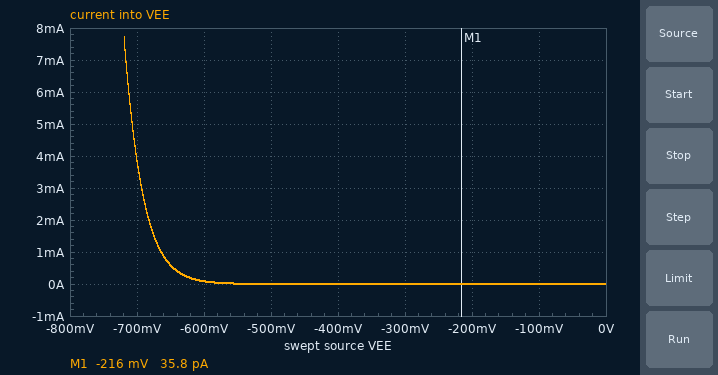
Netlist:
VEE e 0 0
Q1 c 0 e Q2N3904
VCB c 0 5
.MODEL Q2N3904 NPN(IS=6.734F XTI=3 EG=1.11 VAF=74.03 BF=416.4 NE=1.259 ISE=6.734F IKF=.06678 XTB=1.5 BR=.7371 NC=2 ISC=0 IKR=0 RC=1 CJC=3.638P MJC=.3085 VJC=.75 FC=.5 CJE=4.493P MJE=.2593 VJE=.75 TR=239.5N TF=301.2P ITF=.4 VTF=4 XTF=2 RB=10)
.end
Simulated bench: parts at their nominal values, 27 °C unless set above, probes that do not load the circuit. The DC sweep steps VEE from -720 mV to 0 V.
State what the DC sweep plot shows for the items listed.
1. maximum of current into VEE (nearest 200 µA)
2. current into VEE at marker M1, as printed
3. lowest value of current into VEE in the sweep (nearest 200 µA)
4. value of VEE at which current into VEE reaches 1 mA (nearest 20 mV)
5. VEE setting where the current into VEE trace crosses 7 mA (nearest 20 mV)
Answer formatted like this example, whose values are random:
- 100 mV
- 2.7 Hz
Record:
- 7.8 mA
- 35.8 pA
- 0 A
- -660 mV
- -720 mV
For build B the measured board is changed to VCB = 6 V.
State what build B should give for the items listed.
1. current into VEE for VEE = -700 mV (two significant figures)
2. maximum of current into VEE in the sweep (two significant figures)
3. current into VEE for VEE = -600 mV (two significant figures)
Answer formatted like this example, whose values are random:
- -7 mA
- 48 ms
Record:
- 3.9 mA
- 8.0 mA
- 87 µA
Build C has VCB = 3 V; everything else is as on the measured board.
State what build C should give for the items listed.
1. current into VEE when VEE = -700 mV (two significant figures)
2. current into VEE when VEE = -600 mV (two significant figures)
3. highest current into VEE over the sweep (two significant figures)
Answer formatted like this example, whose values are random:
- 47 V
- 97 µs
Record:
- 3.8 mA
- 84 µA
- 7.7 mA
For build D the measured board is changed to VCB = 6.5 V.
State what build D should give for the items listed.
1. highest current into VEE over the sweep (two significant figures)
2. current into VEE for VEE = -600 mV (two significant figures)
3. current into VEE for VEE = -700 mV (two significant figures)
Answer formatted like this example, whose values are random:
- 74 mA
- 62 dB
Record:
- 8.0 mA
- 88 µA
- 3.9 mA
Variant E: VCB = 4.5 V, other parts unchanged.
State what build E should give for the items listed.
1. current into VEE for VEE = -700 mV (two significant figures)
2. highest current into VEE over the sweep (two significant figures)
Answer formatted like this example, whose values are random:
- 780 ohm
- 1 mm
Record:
- 3.8 mA
- 7.8 mA
